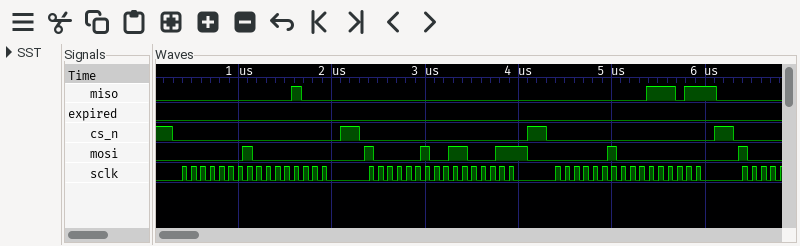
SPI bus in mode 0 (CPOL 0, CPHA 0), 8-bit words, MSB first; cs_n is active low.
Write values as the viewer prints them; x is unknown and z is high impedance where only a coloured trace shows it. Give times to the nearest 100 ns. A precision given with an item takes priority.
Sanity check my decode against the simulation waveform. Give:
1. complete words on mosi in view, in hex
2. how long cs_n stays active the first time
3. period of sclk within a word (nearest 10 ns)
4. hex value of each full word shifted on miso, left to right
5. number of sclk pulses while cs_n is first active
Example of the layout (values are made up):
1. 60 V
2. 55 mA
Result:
1. 01, 00, 82, 63, 02, 00
2. 1800 ns
3. 100 ns
4. 00, 08, 00, 00, 00, 3B
5. 16
